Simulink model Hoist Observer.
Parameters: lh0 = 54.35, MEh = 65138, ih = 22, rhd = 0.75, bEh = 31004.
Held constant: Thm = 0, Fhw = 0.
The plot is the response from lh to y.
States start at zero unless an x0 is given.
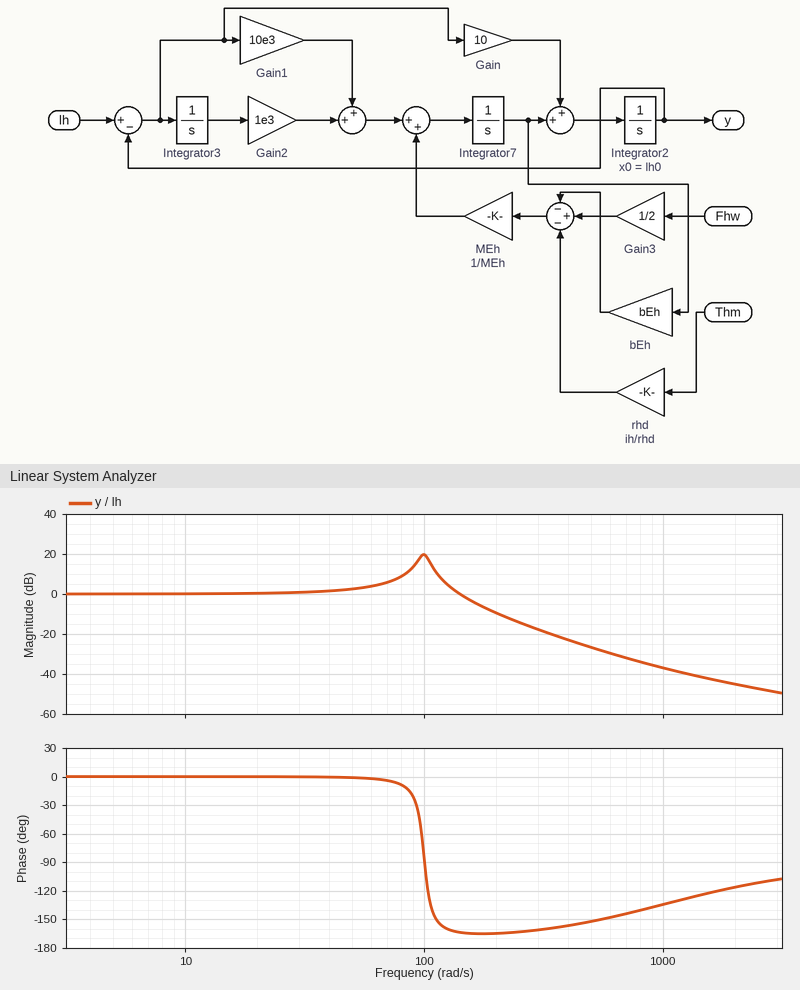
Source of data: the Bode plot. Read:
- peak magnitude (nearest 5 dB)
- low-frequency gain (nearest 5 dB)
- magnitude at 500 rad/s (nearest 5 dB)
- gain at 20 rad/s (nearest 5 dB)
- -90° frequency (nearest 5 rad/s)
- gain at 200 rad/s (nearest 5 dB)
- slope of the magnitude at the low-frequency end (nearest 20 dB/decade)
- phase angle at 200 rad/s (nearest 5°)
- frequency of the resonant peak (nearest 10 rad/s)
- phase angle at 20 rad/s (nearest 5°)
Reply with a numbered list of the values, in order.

1. 20 dB
2. 0 dB
3. -25 dB
4. 0 dB
5. 100 rad/s
6. -10 dB
7. 0 dB/decade
8. -165°
9. 100 rad/s
10. 0°
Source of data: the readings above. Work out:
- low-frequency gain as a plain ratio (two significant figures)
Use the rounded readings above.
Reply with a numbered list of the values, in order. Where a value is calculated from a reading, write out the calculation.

1. 10^(0 / 20) = 1.0
